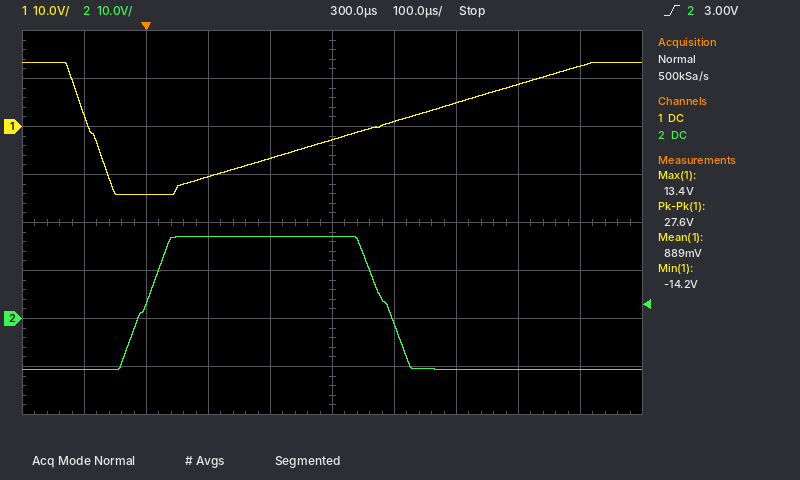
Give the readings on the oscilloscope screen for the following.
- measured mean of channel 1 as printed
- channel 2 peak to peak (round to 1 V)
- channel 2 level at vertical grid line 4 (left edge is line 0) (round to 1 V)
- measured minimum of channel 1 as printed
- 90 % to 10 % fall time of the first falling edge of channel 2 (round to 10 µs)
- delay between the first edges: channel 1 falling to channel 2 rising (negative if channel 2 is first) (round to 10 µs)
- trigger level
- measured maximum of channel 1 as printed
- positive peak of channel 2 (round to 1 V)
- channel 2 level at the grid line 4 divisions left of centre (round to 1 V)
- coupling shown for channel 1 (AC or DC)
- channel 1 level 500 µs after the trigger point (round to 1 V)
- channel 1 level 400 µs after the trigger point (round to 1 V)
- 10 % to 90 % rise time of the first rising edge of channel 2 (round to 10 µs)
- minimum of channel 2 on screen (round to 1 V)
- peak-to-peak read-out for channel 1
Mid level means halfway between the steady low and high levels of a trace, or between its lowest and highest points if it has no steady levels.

889 mV
28 V
17 V
-14.2 V
70 µs
+90 µs
3.00 V
13.4 V
17 V
-11 V
DC
5 V
1 V
70 µs
-11 V
27.6 V
